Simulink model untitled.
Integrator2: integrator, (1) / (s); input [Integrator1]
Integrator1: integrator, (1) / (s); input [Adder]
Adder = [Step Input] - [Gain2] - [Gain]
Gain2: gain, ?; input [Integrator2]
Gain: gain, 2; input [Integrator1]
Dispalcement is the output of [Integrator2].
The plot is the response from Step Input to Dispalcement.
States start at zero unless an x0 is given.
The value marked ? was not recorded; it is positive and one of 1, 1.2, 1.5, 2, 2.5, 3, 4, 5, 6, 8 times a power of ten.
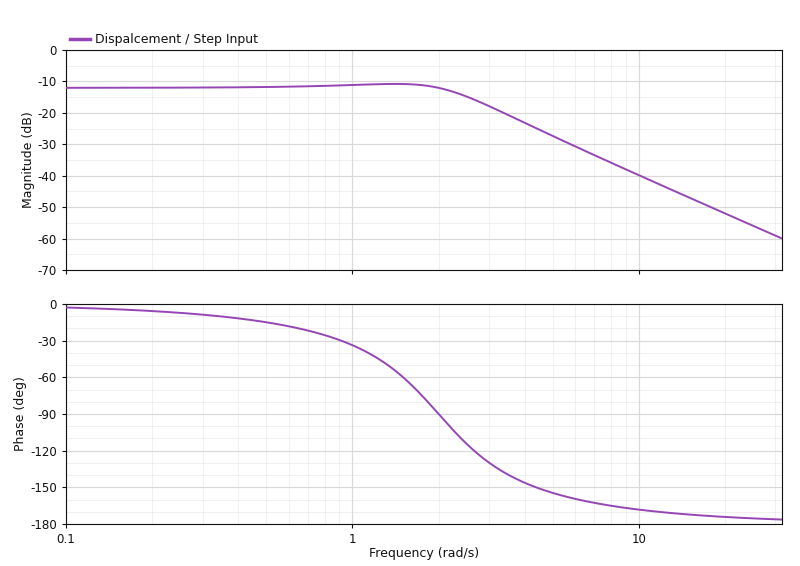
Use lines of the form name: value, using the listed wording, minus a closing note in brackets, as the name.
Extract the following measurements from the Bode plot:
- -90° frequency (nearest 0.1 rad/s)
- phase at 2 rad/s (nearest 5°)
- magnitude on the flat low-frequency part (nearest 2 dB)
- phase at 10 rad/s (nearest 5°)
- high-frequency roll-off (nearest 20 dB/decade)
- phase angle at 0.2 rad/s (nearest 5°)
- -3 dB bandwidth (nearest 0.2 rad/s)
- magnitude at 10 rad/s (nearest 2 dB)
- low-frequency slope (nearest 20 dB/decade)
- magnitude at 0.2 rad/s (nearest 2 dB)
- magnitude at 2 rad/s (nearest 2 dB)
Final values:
-90° frequency: 2.0 rad/s
phase at 2 rad/s: -90°
magnitude on the flat low-frequency part: -12 dB
phase at 10 rad/s: -170°
high-frequency roll-off: -40 dB/decade
phase angle at 0.2 rad/s: -5°
-3 dB bandwidth: 2.6 rad/s
magnitude at 10 rad/s: -40 dB
low-frequency slope: 0 dB/decade
magnitude at 0.2 rad/s: -12 dB
magnitude at 2 rad/s: -12 dB
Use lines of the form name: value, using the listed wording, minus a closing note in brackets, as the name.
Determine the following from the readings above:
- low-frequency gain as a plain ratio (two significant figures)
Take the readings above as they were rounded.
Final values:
low-frequency gain as a plain ratio: 0.25
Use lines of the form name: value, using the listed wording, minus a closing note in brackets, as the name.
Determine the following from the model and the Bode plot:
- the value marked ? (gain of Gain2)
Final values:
the value marked ?: 4
